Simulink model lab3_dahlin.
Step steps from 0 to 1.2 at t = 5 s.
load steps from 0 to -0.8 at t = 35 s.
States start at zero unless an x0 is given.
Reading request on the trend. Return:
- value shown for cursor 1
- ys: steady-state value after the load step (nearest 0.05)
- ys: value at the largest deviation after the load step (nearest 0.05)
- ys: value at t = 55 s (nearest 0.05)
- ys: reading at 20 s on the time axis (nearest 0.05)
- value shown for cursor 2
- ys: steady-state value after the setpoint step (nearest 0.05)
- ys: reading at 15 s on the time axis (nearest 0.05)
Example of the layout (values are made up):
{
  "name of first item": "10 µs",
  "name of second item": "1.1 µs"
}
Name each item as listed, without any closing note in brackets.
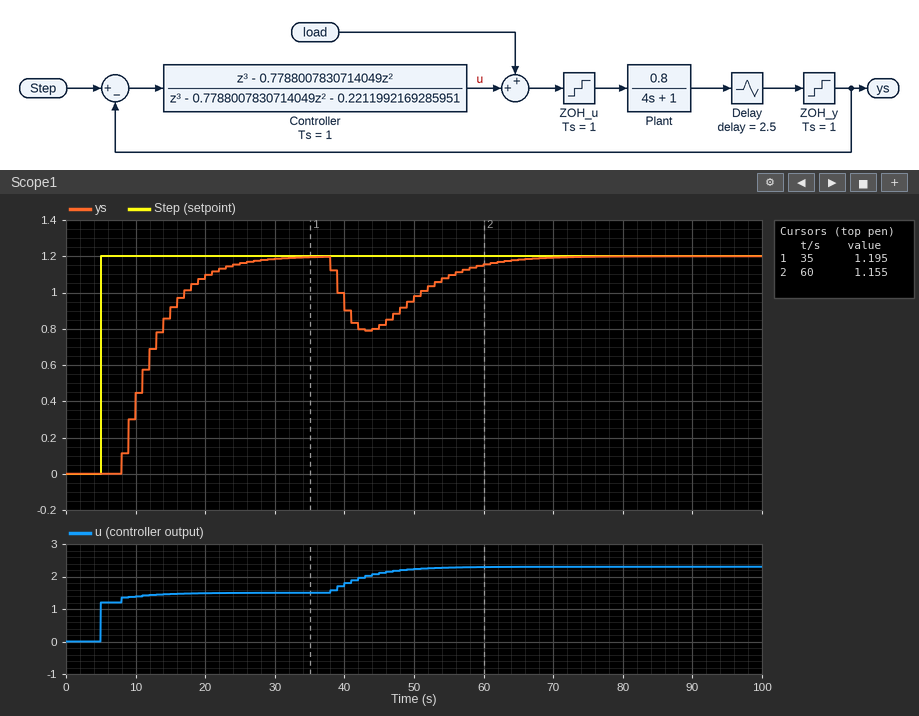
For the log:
{
  "value shown for cursor 1": "1.195",
  "ys: steady-state value after the load step": "1.20",
  "ys: value at the largest deviation after the load step": "0.80",
  "ys: value at t = 55 s": "1.10",
  "ys: reading at 20 s on the time axis": "1.10",
  "value shown for cursor 2": "1.155",
  "ys: steady-state value after the setpoint step": "1.20",
  "ys: reading at 15 s on the time axis": "0.90"
}
